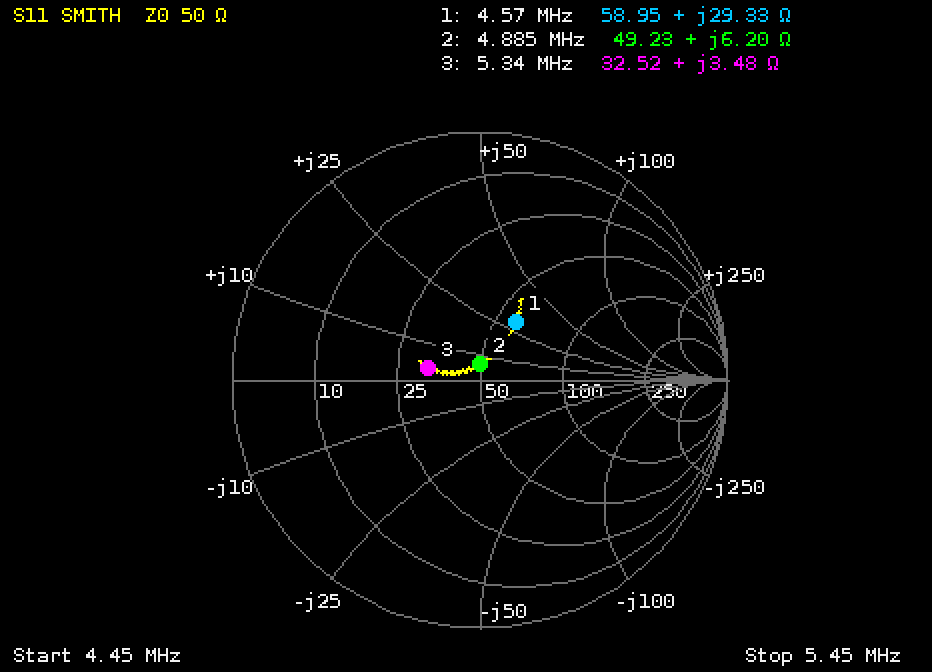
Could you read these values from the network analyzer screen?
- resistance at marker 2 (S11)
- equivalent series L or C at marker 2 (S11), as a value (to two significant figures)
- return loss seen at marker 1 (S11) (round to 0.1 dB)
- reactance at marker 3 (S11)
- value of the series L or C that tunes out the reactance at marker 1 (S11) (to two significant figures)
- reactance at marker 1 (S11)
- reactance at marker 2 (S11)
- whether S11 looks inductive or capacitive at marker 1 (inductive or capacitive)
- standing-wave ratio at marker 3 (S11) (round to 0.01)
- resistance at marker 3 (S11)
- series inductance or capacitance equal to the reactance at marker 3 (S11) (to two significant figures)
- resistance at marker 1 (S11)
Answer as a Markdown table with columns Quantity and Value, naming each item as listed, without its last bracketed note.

| Quantity | Value |
|---|---|
| resistance at marker 2 | 49.23 Ω |
| equivalent series L or C at marker 2 (S11), as a value | 200 nH |
| return loss seen at marker 1 (S11) | 11.3 dB |
| reactance at marker 3 | +3.48 Ω |
| value of the series L or C that tunes out the reactance at marker 1 (S11) | 1.2 nF |
| reactance at marker 1 | +29.33 Ω |
| reactance at marker 2 | +6.20 Ω |
| whether S11 looks inductive or capacitive at marker 1 | inductive |
| standing-wave ratio at marker 3 (S11) | 1.55 |
| resistance at marker 3 | 32.52 Ω |
| series inductance or capacitance equal to the reactance at marker 3 (S11) | 100 nH |
| resistance at marker 1 | 58.95 Ω |
